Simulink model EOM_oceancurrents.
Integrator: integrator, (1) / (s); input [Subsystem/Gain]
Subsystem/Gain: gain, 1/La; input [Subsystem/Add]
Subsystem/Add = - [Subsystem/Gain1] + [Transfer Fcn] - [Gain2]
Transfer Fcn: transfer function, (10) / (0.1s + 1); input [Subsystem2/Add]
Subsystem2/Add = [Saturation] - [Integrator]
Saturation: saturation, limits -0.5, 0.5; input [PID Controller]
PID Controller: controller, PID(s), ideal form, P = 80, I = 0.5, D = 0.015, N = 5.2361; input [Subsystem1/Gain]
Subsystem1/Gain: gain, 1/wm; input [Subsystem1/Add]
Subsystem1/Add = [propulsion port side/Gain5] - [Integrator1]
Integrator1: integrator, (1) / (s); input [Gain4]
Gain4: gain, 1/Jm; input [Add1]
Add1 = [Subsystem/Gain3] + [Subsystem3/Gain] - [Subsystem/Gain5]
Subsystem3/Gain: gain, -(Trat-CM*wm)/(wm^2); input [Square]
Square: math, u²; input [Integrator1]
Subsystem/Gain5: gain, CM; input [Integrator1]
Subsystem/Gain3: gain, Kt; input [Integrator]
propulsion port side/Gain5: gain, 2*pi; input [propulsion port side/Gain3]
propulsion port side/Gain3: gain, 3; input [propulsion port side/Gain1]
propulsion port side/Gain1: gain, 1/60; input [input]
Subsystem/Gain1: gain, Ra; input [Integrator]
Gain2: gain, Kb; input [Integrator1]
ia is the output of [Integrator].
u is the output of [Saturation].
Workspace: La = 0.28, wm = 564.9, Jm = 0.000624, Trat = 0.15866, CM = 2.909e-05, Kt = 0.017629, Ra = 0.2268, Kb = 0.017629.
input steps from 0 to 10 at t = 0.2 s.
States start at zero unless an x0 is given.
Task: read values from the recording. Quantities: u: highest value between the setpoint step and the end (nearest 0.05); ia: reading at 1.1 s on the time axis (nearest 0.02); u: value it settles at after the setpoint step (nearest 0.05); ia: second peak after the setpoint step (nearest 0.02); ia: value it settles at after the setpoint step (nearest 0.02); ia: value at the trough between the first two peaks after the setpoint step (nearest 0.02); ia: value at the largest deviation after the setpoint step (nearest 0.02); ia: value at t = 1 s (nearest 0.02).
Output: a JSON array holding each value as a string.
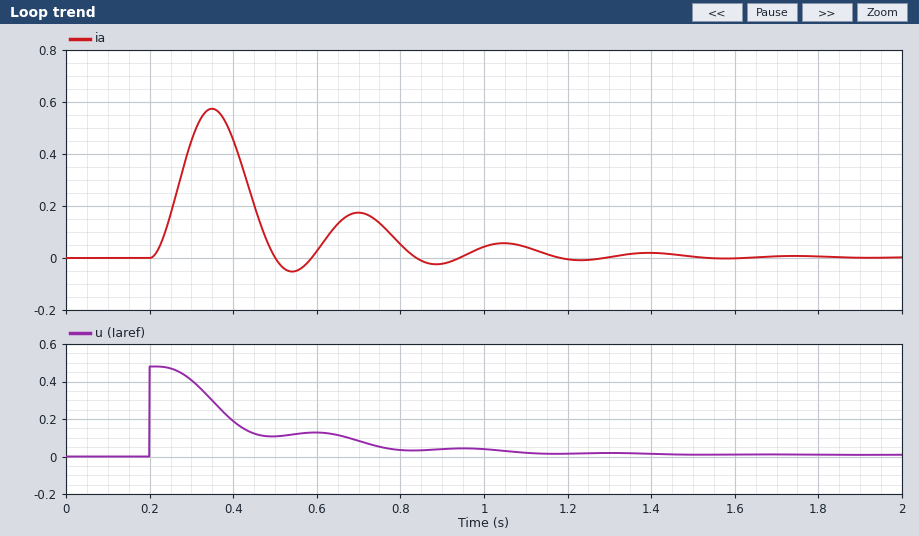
["0.50", "0.04", "0.00", "0.18", "0.00", "-0.06", "0.58", "0.04"]
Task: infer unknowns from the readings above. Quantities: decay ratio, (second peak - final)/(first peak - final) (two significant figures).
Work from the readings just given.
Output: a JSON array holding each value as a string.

["0.31"]
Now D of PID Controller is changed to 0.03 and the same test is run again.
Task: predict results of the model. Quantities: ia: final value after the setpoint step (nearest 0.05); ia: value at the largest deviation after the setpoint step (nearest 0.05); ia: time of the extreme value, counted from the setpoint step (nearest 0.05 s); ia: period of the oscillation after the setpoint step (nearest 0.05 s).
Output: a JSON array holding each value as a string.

["0.00", "0.60", "0.15 s", "0.35 s"]
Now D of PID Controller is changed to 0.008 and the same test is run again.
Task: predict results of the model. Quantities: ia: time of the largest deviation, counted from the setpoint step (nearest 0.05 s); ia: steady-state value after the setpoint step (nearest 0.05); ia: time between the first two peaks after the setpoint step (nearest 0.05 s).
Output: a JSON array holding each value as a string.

["0.15 s", "0.00", "0.35 s"]
